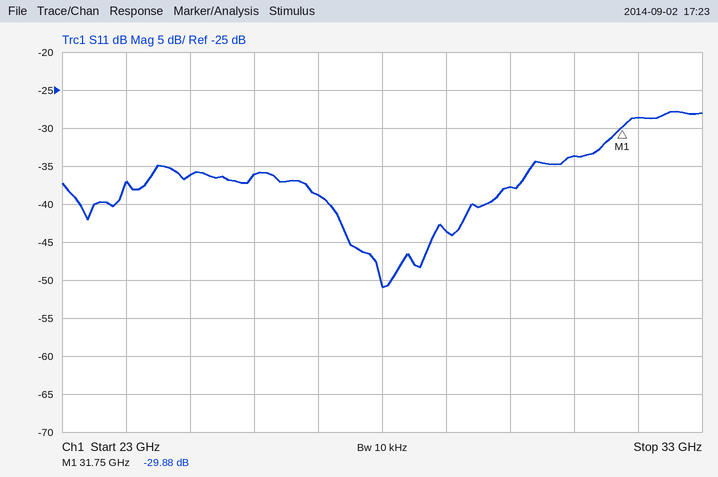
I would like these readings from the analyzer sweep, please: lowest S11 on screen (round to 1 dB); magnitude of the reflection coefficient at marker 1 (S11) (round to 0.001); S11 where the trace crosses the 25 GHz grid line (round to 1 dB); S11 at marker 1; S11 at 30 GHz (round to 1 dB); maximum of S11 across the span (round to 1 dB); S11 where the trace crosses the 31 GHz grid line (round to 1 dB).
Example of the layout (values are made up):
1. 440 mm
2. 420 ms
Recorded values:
1. -51 dB
2. 0.032
3. -36 dB
4. -29.88 dB
5. -38 dB
6. -28 dB
7. -34 dB
